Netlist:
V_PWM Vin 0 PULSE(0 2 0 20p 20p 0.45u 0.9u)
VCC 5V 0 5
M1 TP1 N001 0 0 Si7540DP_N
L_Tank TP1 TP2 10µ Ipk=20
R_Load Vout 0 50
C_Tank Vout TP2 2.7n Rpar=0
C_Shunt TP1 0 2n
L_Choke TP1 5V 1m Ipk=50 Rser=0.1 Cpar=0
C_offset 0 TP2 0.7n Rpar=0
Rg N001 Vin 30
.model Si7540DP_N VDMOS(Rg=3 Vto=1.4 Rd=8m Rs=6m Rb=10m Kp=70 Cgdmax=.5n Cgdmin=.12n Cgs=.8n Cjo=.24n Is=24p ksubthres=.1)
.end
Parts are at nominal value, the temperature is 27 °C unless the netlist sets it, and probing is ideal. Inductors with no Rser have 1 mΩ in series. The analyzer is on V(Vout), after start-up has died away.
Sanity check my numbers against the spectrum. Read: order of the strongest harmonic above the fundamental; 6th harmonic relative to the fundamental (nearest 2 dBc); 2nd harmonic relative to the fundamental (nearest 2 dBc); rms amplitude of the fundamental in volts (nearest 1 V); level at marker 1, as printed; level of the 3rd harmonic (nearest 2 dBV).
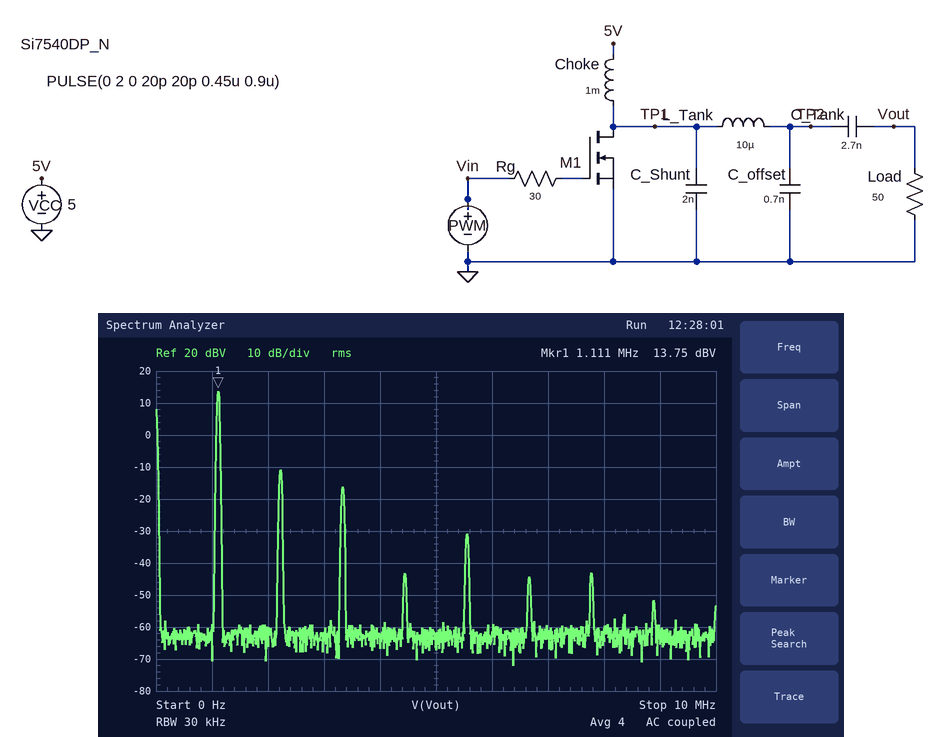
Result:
2
-58 dBc
-24 dBc
5 V
13.75 dBV
-16 dBV
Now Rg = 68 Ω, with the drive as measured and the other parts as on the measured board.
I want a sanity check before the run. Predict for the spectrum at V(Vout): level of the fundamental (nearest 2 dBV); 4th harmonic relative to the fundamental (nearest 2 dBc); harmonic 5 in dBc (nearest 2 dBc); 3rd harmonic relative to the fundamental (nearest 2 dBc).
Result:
12 dBV
-46 dBc
-52 dBc
-32 dBc
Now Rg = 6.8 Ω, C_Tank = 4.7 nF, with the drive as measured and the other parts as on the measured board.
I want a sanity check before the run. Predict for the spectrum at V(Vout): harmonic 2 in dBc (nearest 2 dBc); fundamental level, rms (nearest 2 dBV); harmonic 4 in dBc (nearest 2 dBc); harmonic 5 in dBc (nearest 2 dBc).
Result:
-20 dBc
12 dBV
-38 dBc
-40 dBc
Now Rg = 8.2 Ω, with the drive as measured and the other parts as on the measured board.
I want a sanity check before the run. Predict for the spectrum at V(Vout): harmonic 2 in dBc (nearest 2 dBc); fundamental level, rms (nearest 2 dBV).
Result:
-22 dBc
14 dBV
